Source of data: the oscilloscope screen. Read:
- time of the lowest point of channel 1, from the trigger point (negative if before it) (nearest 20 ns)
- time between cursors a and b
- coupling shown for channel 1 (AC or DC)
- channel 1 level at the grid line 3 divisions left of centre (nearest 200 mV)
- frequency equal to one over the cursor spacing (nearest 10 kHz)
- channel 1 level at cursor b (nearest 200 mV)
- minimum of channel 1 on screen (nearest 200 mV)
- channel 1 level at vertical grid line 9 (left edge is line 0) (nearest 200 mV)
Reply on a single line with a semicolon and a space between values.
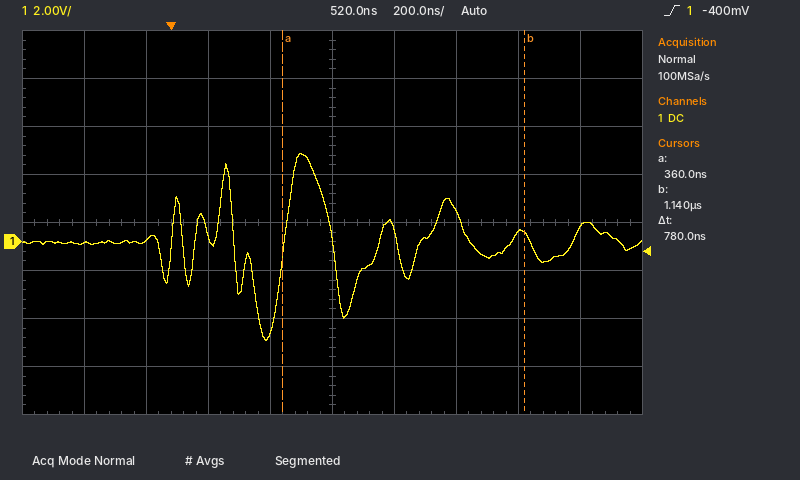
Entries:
+300 ns; 780 ns; DC; 0.0 V; 1.28 MHz; 400 mV; -4.2 V; 600 mV
